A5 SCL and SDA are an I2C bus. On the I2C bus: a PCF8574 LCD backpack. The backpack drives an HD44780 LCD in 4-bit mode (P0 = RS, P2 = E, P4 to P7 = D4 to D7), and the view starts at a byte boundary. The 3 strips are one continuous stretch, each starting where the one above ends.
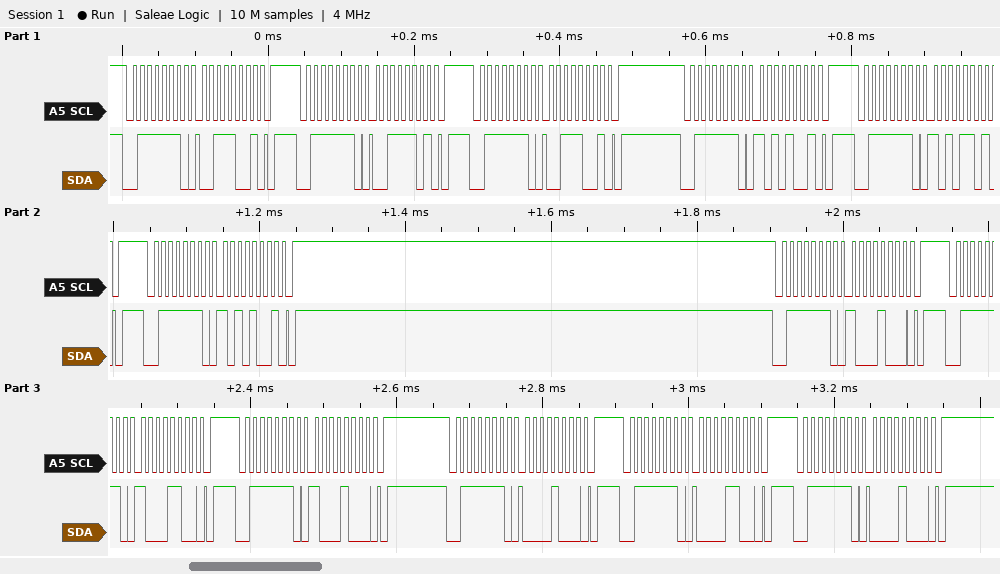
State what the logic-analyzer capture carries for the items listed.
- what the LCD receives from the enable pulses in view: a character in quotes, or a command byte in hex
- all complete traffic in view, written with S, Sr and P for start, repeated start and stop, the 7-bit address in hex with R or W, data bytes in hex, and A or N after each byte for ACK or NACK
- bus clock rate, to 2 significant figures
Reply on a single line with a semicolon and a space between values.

':' 0x80; S 3FW A 39 A P S 3FW A 3D A P S 3FW A 39 A P S 3FW A A9 A P S 3FW A AD A P S 3FW A A9 A P S 3FW A 88 A P S 3FW A 8C A P S 3FW A 88 A P S 3FW A 08 A P S 3FW A 0C A P S 3FW A 08 A P; 100 kHz
